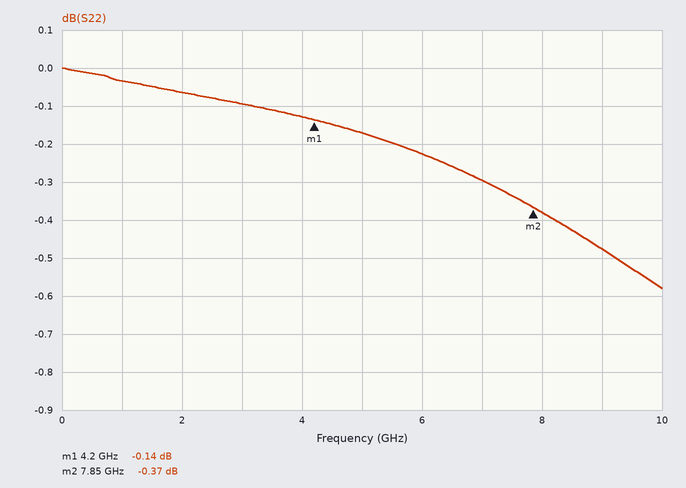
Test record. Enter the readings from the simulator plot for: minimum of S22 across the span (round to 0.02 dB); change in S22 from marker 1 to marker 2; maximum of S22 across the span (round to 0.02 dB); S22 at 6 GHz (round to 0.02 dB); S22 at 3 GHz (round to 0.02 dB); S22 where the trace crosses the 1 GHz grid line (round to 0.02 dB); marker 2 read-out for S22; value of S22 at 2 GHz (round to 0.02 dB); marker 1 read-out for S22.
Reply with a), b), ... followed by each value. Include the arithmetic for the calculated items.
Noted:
a) -0.58 dB
b) -0.37 − (-0.14) = -0.23 dB
c) 0.00 dB
d) -0.22 dB
e) -0.10 dB
f) -0.04 dB
g) -0.37 dB
h) -0.06 dB
i) -0.14 dB
